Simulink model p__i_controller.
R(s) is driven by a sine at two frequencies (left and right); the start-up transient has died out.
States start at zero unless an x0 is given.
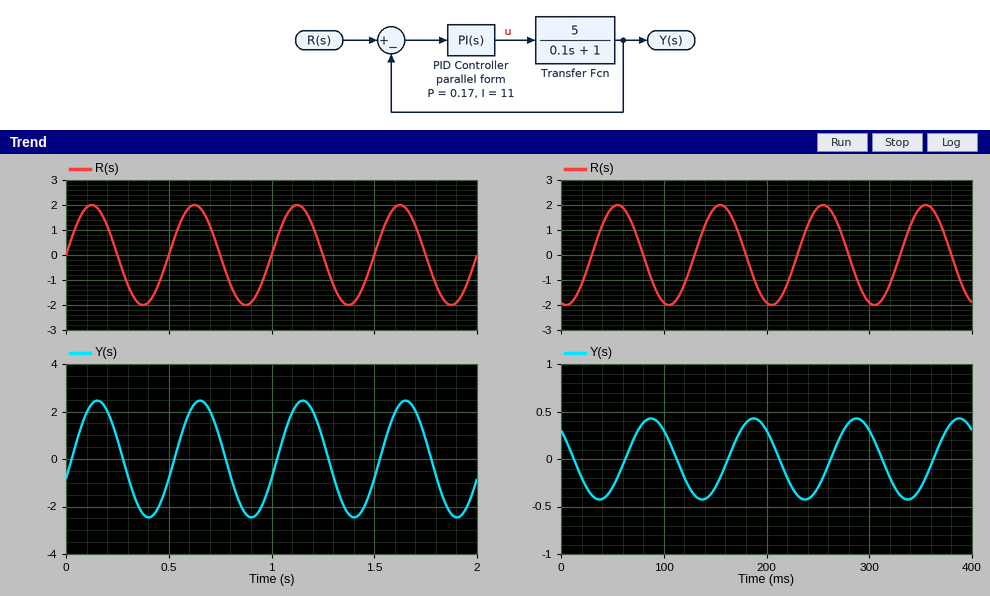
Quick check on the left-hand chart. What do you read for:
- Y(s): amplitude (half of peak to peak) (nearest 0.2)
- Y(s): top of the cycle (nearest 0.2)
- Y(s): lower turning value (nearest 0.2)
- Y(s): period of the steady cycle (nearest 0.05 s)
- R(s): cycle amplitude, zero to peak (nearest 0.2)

2.4
2.4
-2.4
0.50 s
2.0
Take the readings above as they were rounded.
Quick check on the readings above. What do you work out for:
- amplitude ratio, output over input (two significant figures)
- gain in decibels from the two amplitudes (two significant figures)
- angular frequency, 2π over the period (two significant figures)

1.2
1.6 dB
13 rad/s
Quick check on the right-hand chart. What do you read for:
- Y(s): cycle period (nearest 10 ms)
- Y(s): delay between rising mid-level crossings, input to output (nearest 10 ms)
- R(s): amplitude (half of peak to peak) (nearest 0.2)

100 ms
30 ms
2.0
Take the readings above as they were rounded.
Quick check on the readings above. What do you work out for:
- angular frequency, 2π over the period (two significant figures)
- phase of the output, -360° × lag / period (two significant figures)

0.063 rad/ms
-110°
